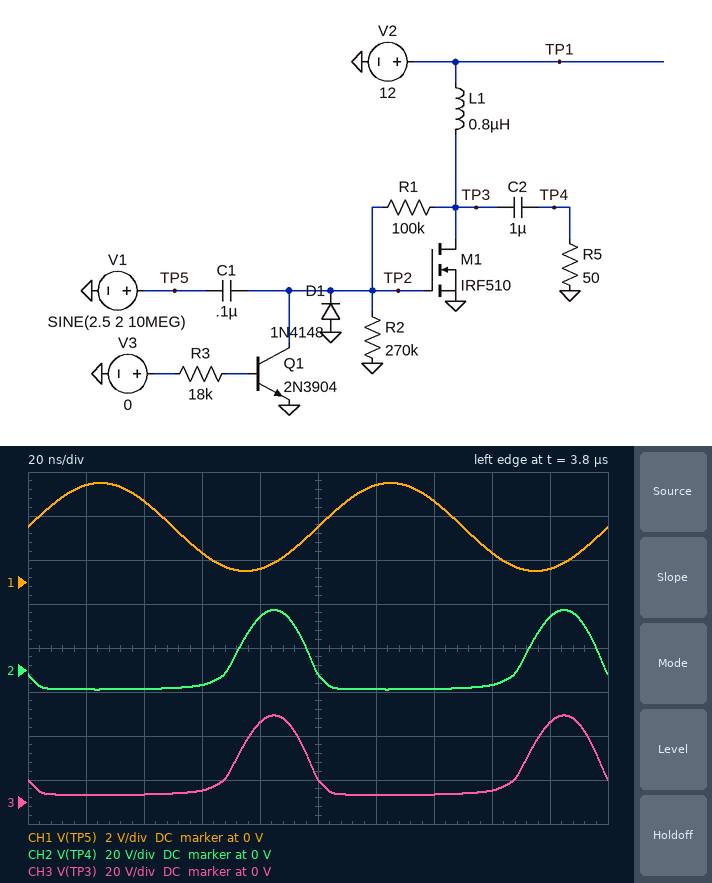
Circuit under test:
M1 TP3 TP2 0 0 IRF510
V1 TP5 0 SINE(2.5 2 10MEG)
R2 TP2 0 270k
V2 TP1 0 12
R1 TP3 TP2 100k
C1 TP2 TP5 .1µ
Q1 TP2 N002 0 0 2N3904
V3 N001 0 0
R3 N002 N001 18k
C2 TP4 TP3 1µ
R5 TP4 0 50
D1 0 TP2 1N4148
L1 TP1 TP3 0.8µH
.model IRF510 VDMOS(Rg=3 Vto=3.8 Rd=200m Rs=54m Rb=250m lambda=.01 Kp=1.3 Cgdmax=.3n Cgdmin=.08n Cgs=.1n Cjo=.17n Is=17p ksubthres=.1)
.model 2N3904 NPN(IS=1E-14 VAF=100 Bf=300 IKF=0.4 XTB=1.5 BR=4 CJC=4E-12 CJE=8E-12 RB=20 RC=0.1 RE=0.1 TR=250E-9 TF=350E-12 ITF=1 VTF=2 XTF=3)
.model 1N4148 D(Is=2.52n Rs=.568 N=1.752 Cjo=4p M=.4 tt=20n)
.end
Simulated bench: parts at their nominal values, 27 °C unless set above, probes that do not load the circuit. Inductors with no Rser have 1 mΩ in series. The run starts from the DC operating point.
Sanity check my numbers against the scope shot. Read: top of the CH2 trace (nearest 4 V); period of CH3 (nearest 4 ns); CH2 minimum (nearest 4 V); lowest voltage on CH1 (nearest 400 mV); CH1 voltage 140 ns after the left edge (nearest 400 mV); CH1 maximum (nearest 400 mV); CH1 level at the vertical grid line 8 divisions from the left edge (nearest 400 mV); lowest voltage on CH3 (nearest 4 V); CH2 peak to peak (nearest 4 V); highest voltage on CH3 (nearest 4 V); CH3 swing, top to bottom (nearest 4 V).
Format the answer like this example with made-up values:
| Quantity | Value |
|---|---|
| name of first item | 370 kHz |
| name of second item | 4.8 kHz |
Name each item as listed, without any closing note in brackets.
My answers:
| Quantity | Value |
|---|---|
| top of the CH2 trace | 28 V |
| period of CH3 | 100 ns |
| CH2 minimum | -8 V |
| lowest voltage on CH1 | 400 mV |
| CH1 voltage 140 ns after the left edge | 3.6 V |
| CH1 maximum | 4.4 V |
| CH1 level at the vertical grid line 8 divisions from the left edge | 1.2 V |
| lowest voltage on CH3 | 4 V |
| CH2 peak to peak | 36 V |
| highest voltage on CH3 | 40 V |
| CH3 swing, top to bottom | 36 V |
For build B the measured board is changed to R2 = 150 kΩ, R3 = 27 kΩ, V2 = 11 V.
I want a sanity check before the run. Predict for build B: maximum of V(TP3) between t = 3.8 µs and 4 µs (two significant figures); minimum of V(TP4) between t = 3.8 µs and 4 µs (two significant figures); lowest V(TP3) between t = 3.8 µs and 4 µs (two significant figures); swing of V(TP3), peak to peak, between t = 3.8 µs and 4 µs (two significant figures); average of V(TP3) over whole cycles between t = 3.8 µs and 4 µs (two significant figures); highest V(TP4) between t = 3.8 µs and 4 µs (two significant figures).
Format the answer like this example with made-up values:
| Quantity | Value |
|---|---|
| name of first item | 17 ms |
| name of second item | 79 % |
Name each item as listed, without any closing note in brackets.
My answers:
| Quantity | Value |
|---|---|
| maximum of V(TP3) between t = 3.8 µs and 4 µs | 42 V |
| minimum of V(TP4) between t = 3.8 µs and 4 µs | -10 V |
| lowest V(TP3) between t = 3.8 µs and 4 µs | 820 mV |
| swing of V(TP3), peak to peak, between t = 3.8 µs and 4 µs | 41 V |
| average of V(TP3) over whole cycles between t = 3.8 µs and 4 µs | 11 V |
| highest V(TP4) between t = 3.8 µs and 4 µs | 31 V |
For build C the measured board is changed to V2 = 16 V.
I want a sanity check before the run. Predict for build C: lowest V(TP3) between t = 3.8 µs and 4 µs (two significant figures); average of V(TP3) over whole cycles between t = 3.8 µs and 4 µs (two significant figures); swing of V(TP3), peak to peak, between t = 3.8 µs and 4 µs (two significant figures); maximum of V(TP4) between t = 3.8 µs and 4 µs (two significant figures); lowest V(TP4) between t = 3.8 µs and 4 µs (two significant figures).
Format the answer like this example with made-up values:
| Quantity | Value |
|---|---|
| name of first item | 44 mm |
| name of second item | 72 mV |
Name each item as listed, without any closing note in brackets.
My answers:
| Quantity | Value |
|---|---|
| lowest V(TP3) between t = 3.8 µs and 4 µs | 8.0 V |
| average of V(TP3) over whole cycles between t = 3.8 µs and 4 µs | 16 V |
| swing of V(TP3), peak to peak, between t = 3.8 µs and 4 µs | 32 V |
| maximum of V(TP4) between t = 3.8 µs and 4 µs | 24 V |
| lowest V(TP4) between t = 3.8 µs and 4 µs | -8.1 V |
